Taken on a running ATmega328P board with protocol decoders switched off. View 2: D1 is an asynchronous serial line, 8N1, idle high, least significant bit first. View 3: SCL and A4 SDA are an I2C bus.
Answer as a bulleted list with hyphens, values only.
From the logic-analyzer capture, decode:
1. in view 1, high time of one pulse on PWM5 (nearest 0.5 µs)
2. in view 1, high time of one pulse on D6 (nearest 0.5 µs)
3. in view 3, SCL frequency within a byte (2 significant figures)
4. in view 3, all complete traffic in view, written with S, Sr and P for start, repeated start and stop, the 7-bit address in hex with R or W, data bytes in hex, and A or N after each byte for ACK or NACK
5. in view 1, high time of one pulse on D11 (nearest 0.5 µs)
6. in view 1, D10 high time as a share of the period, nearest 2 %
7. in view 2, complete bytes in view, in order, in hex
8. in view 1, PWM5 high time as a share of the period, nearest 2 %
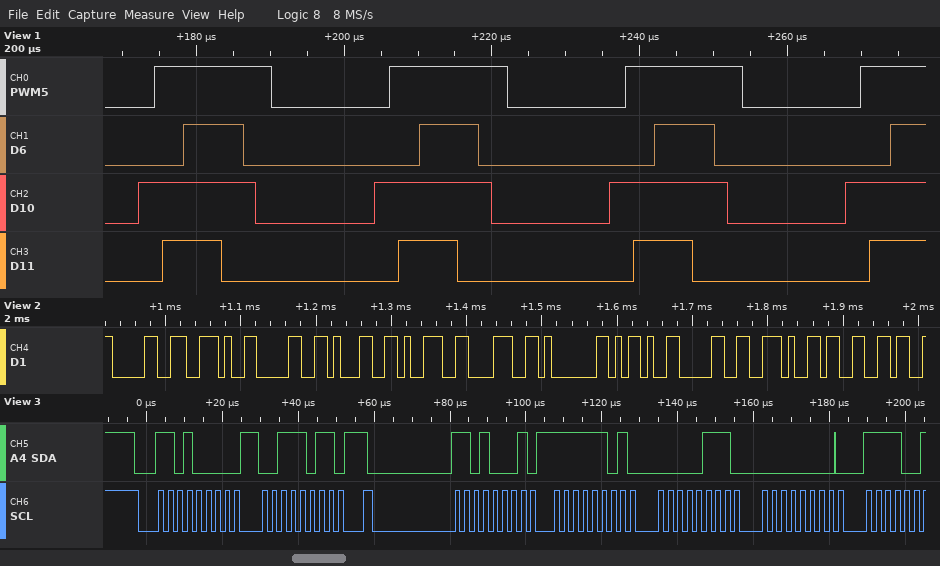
- 16.0 µs
- 8.0 µs
- 400 kHz
- S 68W A 3B A Sr 68R A FD A 07 A 00 A
- 8.0 µs
- 50 %
- 30 2E 30 31 39 38 01 2D 30 2E 33
- 50 %
